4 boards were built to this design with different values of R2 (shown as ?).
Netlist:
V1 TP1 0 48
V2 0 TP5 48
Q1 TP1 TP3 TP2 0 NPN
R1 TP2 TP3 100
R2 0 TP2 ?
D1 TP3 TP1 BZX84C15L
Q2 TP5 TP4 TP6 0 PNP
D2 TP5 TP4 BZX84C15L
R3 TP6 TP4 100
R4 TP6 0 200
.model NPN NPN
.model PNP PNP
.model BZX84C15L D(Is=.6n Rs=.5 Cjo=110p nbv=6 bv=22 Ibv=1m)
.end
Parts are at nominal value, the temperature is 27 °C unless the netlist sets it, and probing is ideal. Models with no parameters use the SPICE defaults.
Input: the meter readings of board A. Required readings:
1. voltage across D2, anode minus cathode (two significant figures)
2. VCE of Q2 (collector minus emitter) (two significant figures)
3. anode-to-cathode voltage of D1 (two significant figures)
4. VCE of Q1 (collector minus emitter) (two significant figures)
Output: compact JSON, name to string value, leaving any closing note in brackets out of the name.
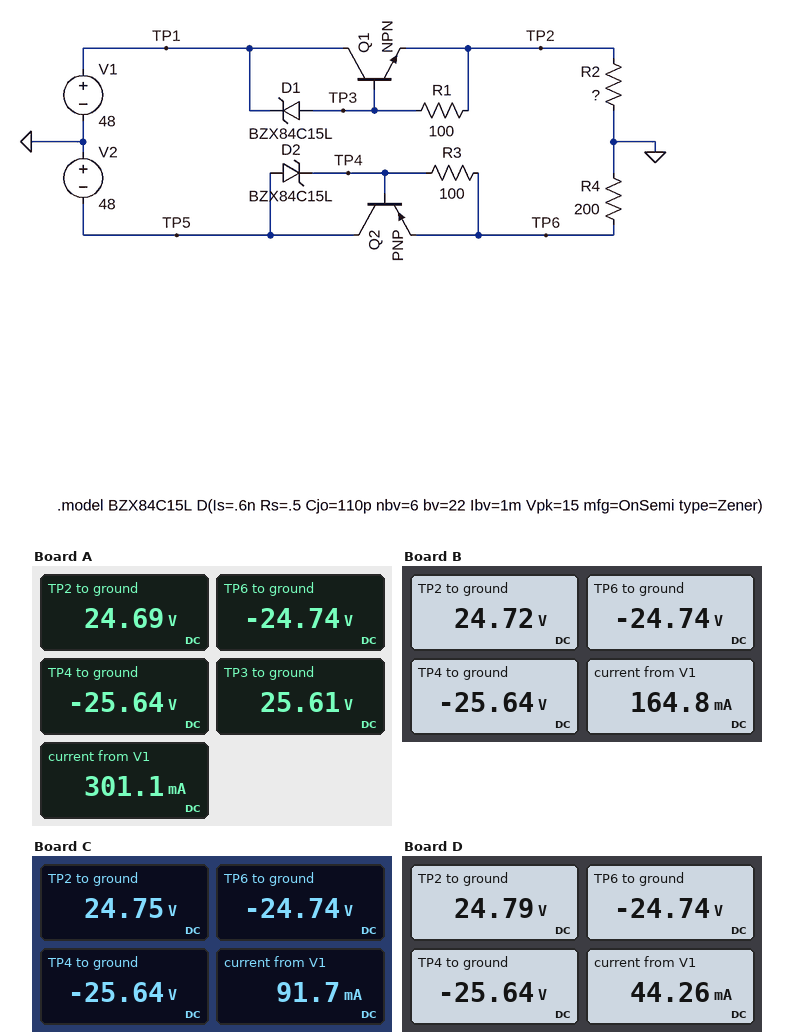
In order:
{"voltage across D2, anode minus cathode": "-22 V", "VCE of Q2 (collector minus emitter)": "-23 V", "anode-to-cathode voltage of D1": "-22 V", "VCE of Q1 (collector minus emitter)": "23 V"}
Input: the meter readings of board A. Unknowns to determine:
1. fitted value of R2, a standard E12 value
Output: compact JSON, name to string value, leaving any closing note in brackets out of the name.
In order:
{"fitted value of R2, a standard E12 value": "82 Ω"}
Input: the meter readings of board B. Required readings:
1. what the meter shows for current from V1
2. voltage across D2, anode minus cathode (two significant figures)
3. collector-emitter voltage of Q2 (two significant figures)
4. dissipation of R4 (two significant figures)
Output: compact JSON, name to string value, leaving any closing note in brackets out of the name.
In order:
{"what the meter shows for current from V1": "164.8 mA", "voltage across D2, anode minus cathode": "-22 V", "collector-emitter voltage of Q2": "-23 V", "dissipation of R4": "3.1 W"}
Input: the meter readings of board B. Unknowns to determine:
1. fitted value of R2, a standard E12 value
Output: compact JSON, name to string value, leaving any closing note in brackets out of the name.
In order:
{"fitted value of R2, a standard E12 value": "150 Ω"}
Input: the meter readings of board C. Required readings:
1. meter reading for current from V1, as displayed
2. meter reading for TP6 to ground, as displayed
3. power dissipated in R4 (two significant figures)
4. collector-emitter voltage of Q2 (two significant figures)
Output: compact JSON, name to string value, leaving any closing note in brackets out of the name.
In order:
{"meter reading for current from V1, as displayed": "91.7 mA", "meter reading for TP6 to ground, as displayed": "-24.74 V", "power dissipated in R4": "3.1 W", "collector-emitter voltage of Q2": "-23 V"}
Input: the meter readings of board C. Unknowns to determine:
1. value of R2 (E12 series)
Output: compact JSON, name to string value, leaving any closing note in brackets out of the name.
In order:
{"value of R2": "270 Ω"}
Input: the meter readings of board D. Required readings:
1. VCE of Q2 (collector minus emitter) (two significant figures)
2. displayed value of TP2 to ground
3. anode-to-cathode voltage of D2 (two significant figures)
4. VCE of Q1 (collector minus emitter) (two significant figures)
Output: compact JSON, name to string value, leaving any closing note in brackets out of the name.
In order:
{"VCE of Q2 (collector minus emitter)": "-23 V", "displayed value of TP2 to ground": "24.79 V", "anode-to-cathode voltage of D2": "-22 V", "VCE of Q1 (collector minus emitter)": "23 V"}
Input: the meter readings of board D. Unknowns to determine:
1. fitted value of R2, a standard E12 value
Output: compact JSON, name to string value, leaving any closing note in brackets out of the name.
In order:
{"fitted value of R2, a standard E12 value": "560 Ω"}
